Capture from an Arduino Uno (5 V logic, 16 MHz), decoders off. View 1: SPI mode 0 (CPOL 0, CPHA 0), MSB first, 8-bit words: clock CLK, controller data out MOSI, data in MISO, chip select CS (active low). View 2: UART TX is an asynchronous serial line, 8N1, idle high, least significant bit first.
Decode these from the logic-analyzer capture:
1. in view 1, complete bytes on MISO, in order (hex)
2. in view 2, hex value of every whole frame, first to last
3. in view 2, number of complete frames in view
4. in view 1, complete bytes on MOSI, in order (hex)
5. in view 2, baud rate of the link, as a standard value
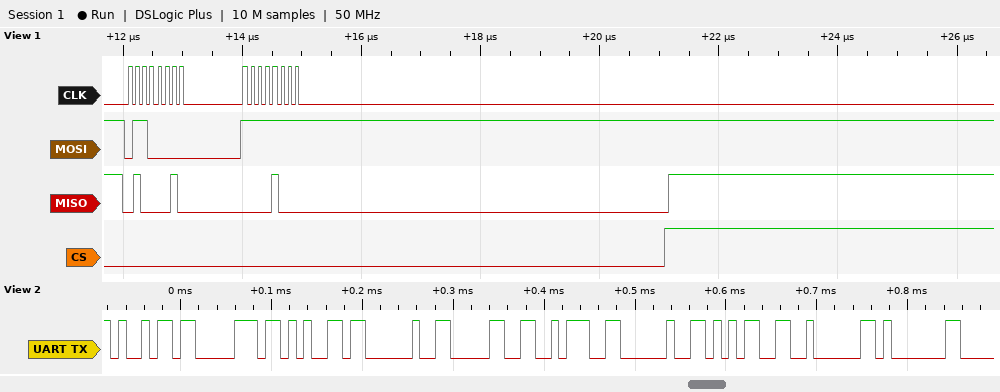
42 08
0x69 0x70 0x65 0x20 0x30 0x3A 0x20 0x35 0x02 0x01
10
60 FF
115200 baud
